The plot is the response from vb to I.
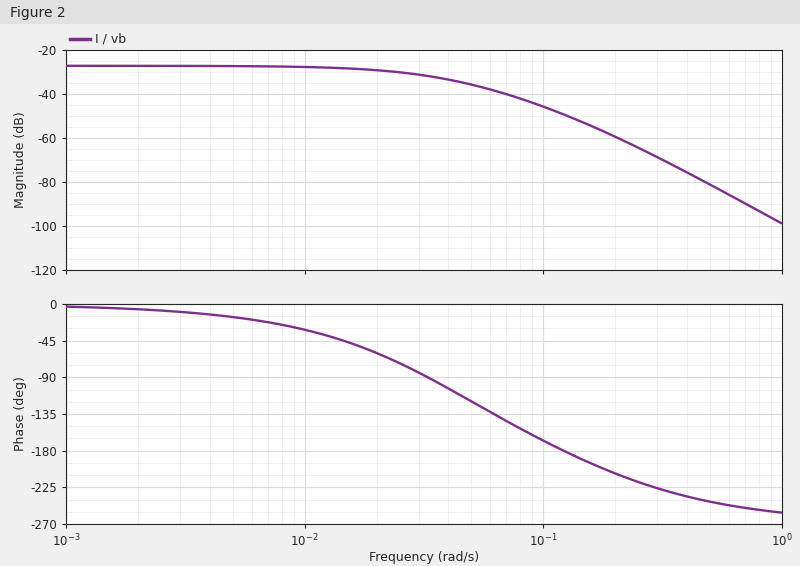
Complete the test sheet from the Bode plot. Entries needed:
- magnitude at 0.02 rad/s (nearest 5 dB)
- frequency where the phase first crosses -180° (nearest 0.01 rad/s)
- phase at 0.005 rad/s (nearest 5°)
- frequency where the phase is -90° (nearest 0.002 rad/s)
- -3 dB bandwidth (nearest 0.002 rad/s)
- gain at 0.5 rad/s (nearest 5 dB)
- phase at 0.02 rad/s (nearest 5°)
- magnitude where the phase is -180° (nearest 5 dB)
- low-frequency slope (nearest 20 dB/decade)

-30 dB
0.12 rad/s
-15°
0.032 rad/s
0.026 rad/s
-80 dB
-60°
-50 dB
0 dB/decade
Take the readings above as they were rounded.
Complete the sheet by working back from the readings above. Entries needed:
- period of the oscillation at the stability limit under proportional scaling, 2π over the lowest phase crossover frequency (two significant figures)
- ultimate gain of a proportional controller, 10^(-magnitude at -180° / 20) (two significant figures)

52 s
320
